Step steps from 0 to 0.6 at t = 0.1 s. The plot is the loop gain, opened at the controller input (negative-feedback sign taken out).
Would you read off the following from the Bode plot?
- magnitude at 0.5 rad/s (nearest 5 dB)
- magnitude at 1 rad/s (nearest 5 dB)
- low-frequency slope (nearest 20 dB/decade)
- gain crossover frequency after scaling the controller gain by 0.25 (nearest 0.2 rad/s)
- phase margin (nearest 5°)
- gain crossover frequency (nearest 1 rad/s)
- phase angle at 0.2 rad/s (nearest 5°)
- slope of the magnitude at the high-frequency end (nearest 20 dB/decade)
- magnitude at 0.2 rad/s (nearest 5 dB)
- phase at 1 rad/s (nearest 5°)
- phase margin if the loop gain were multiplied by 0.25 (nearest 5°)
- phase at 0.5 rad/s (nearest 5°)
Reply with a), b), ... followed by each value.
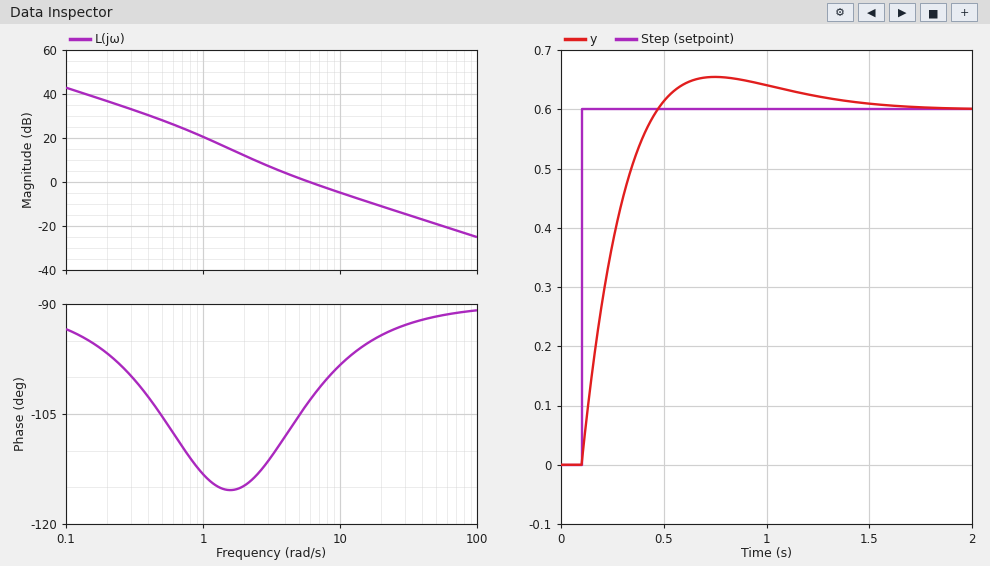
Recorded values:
a) 30 dB
b) 20 dB
c) -20 dB/decade
d) 2.0 rad/s
e) 75°
f) 6 rad/s
g) -95°
h) -20 dB/decade
i) 35 dB
j) -115°
k) 65°
l) -105°
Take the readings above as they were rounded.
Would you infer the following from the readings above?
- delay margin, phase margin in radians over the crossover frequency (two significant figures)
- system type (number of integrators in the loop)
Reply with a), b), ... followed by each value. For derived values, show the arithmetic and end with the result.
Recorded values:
a) 75 × π / 180 / 6 = 0.22 s
b) 1
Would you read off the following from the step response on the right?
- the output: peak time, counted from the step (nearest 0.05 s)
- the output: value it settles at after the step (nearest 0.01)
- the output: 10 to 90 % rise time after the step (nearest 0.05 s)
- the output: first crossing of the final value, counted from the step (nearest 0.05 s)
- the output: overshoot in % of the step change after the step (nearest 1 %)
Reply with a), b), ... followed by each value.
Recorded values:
a) 0.65 s
b) 0.60
c) 0.25 s
d) 0.35 s
e) 9 %
